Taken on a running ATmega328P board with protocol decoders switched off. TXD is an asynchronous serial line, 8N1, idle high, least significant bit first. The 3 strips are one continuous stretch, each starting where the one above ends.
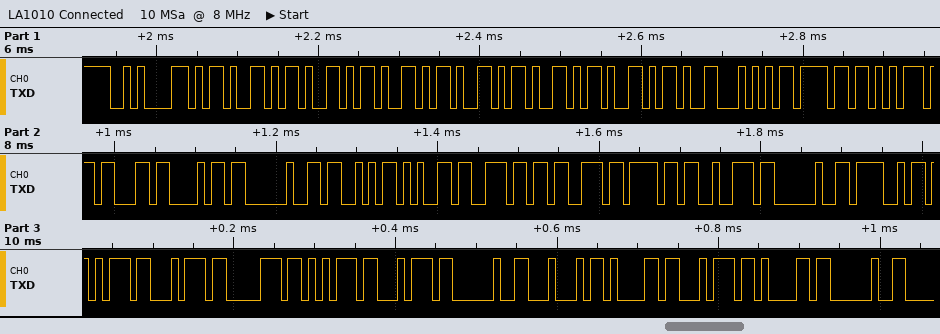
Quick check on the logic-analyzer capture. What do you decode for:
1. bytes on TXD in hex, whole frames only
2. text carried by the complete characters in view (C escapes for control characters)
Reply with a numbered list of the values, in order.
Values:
1. 0A 2D 2D 2D 2D 2D 2D 2D 54 6F 75 63 68 20 53 65 6E 73 6F 72 20 4F 75 74 70 75 74 20 44 61 74 61 20
2. "\n-------Touch Sensor Output Data "
